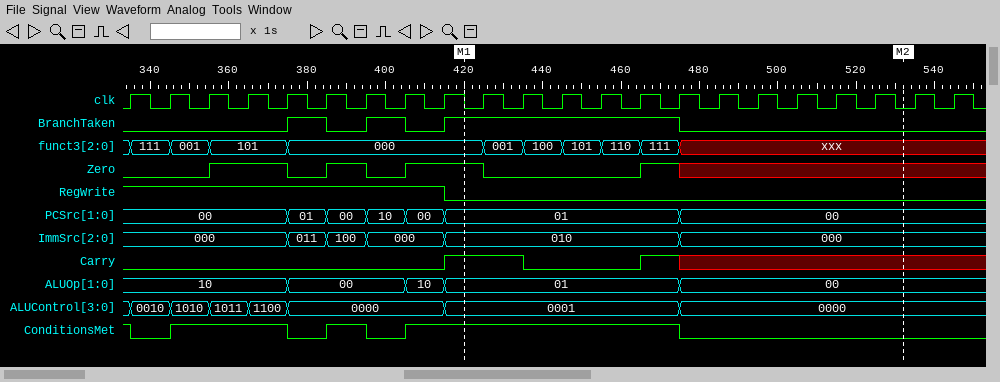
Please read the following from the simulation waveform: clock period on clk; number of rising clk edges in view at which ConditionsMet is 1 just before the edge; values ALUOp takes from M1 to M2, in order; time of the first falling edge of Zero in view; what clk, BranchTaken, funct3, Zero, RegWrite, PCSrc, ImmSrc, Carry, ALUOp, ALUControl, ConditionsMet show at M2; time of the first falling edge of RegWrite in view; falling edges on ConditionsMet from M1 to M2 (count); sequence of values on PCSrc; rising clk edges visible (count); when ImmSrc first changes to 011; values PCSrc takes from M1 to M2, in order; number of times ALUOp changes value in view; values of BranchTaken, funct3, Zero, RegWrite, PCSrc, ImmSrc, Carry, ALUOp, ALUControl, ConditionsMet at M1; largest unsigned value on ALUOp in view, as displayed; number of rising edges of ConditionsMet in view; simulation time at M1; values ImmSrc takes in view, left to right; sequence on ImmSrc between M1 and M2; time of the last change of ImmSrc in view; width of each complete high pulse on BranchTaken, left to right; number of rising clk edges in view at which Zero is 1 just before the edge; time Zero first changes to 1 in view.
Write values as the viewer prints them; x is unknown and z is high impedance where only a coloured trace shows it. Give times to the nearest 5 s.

10 s
12
01, 00
375 s
clk=0, BranchTaken=0, funct3=xxx, Zero=x, RegWrite=0, PCSrc=00, ImmSrc=000, Carry=x, ALUOp=00, ALUControl=0000, ConditionsMet=0
415 s
1
00, 01, 00, 10, 00, 01, 00
22
375 s
01, 00
4
BranchTaken=1, funct3=000, Zero=1, RegWrite=0, PCSrc=01, ImmSrc=010, Carry=1, ALUOp=01, ALUControl=0001, ConditionsMet=1
10
3
420 s
000, 011, 100, 000, 010, 000
010, 000
475 s
10 s, 10 s, 60 s
6
355 s
